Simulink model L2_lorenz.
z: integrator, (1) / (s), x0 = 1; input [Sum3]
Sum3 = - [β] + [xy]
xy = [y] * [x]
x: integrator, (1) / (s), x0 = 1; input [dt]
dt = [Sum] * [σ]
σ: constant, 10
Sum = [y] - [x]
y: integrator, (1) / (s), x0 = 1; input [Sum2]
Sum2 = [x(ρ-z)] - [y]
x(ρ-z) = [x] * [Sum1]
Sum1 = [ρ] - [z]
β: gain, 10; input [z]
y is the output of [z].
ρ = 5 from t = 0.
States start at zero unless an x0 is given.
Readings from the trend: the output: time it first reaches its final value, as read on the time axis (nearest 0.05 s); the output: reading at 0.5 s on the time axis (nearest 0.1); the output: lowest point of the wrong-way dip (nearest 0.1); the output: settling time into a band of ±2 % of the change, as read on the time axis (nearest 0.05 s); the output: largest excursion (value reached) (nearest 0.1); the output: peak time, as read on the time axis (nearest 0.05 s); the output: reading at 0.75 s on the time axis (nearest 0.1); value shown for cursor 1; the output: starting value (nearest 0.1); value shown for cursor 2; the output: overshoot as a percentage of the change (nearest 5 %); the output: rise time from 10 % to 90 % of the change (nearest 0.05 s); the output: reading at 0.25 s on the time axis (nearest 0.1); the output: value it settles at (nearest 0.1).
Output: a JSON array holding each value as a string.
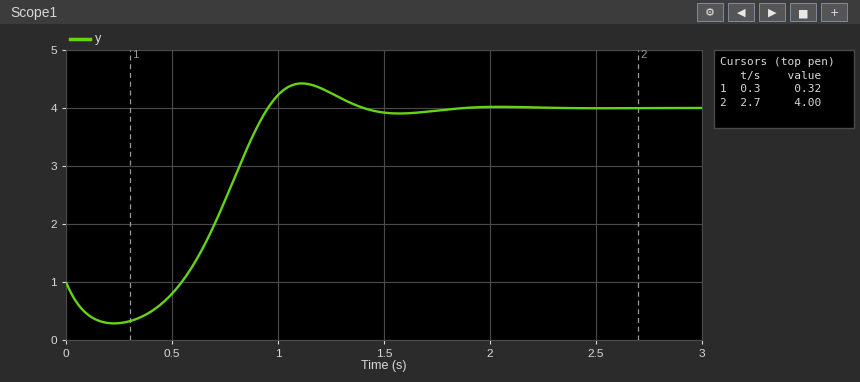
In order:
["0.95 s", "0.8", "0.3", "1.70 s", "4.4", "1.10 s", "2.4", "0.32", "1.0", "4.00", "15 %", "0.30 s", "0.3", "4.0"]
